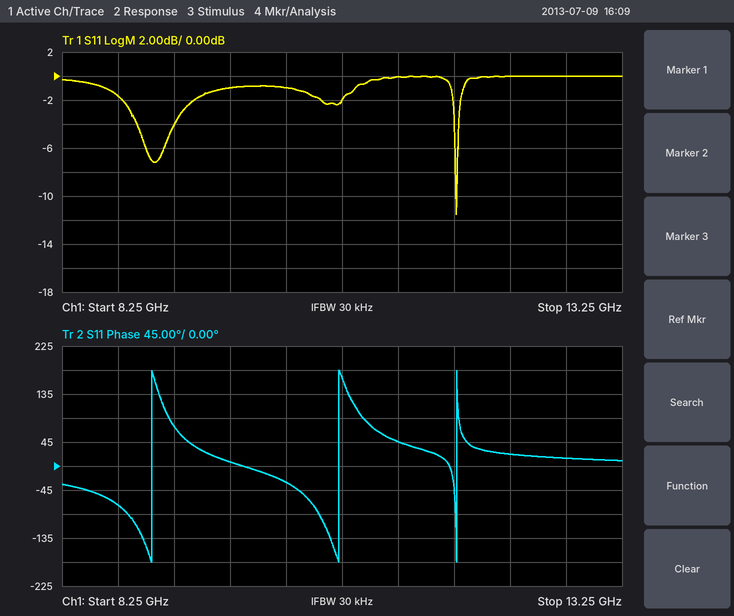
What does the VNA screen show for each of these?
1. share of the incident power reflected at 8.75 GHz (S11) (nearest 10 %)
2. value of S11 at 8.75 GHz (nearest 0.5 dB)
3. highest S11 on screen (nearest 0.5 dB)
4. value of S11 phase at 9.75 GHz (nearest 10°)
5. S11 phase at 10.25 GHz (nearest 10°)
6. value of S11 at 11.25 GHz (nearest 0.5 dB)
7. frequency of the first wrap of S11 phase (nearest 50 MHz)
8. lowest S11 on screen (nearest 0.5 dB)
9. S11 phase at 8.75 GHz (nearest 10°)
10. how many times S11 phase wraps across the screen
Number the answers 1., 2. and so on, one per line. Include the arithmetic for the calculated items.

1. 10^(-1.5/10) ≈ 70.8 %, so 70 % to the nearest 10 %
2. -1.5 dB
3. 0.0 dB
4. 10°
5. -30°
6. 0.0 dB
7. 9.05 GHz
8. -11.5 dB
9. -70°
10. 3
